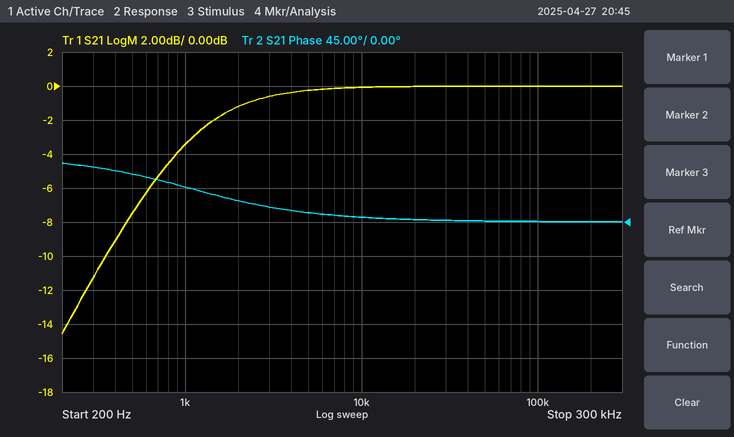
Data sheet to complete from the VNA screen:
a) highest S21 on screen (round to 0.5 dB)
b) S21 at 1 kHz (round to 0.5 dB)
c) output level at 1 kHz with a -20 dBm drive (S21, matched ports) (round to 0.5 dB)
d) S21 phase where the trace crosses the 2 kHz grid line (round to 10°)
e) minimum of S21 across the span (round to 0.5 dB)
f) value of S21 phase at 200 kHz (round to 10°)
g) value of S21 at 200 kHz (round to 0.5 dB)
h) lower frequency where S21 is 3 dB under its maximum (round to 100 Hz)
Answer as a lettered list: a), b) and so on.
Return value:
a) 0.0 dB
b) -3.5 dB
c) -23.5 dBm
d) 30°
e) -14.5 dB
f) 0°
g) 0.0 dB
h) 1.1 kHz
